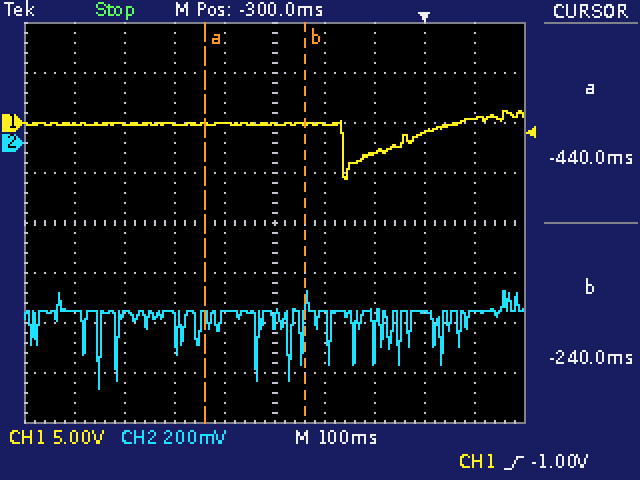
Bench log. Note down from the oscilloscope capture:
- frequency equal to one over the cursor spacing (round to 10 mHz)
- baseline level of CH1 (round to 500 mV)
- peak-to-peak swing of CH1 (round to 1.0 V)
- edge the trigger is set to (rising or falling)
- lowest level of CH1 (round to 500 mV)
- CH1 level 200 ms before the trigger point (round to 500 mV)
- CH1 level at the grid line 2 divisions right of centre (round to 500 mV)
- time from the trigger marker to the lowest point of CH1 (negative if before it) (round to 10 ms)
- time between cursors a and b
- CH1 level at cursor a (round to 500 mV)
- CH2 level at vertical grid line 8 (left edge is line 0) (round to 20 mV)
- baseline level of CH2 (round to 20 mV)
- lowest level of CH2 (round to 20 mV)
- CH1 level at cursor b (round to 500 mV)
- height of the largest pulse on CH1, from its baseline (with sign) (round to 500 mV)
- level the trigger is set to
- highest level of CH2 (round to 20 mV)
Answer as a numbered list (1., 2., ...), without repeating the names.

1. 5.00 Hz
2. 0.0 V
3. 7.0 V
4. rising
5. -5.5 V
6. 0.0 V
7. -3.0 V
8. -160 ms
9. 200 ms
10. 0.0 V
11. -680 mV
12. -680 mV
13. -980 mV
14. 0.0 V
15. -5.5 V
16. -1.00 V
17. -600 mV
